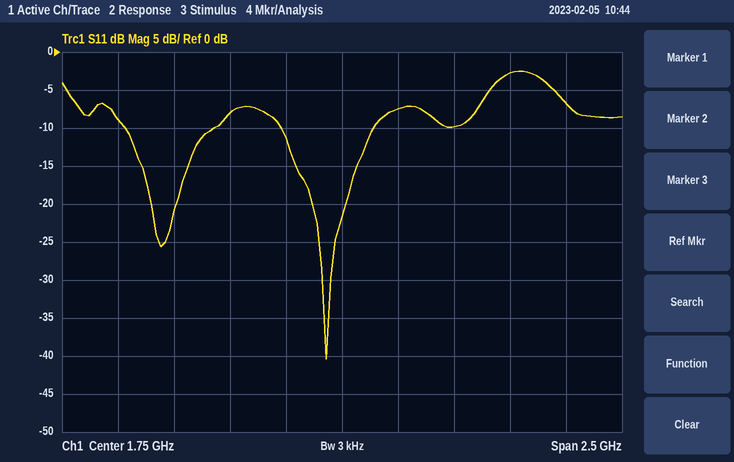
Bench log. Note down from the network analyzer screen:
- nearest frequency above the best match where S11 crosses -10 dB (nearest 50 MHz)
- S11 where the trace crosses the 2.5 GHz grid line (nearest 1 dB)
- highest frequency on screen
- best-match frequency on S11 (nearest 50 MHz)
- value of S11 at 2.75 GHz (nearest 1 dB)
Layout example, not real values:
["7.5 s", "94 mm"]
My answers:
["1.90 GHz", "-3 dB", "3 GHz", "1.70 GHz", "-7 dB"]
